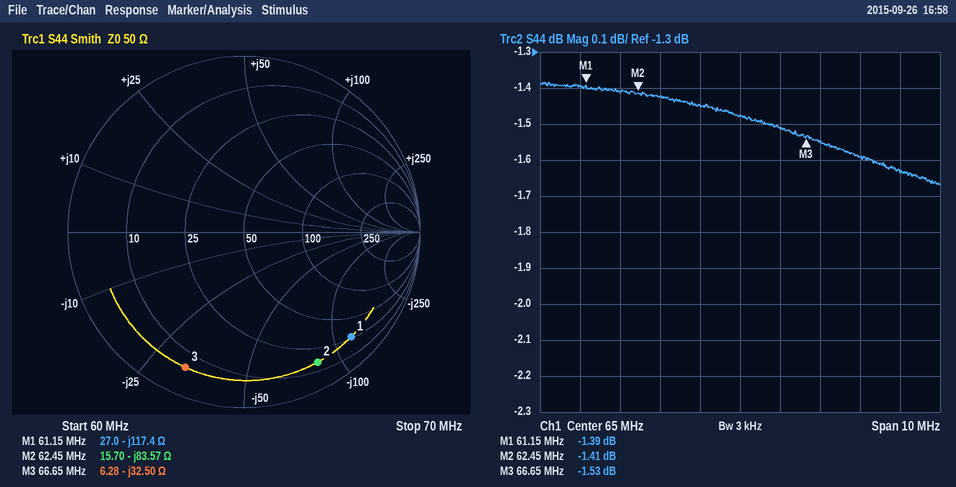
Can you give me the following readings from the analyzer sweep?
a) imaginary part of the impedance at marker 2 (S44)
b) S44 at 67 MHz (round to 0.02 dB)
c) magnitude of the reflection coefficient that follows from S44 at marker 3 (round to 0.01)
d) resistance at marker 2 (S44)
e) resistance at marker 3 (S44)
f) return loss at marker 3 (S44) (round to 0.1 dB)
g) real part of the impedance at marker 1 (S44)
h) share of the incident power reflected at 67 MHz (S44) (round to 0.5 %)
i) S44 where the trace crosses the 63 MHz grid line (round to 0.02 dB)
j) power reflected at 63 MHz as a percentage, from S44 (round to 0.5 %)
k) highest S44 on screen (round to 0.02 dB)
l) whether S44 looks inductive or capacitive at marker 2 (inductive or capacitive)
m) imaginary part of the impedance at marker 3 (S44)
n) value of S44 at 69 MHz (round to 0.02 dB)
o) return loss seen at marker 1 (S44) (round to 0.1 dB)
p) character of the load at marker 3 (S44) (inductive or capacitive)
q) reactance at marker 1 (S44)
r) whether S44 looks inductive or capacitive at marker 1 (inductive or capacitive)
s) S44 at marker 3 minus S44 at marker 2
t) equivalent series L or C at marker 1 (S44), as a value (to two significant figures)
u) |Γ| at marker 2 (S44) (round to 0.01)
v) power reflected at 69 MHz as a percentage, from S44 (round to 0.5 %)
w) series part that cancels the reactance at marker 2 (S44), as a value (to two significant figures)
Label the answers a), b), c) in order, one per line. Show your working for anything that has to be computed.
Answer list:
a) -83.57 Ω
b) -1.54 dB
c) 10^(-1.53/20) ≈ 0.84
d) 15.70 Ω
e) 6.28 Ω
f) 1.5 dB
g) 27.0 Ω
h) 10^(-1.54/10) ≈ 70.1 %, so 70.0 % to the nearest 0.5 %
i) -1.42 dB
j) 10^(-1.42/10) ≈ 72.1 %, so 72.0 % to the nearest 0.5 %
k) -1.38 dB
l) capacitive
m) -32.50 Ω
n) -1.64 dB
o) 1.4 dB
p) capacitive
q) -117.4 Ω
r) capacitive
s) -1.53 − (-1.41) = -0.12 dB
t) C = 1/(2π × 61.15 MHz × 117.4 Ω) ≈ 22 pF
u) 0.85
v) 10^(-1.64/10) ≈ 68.5 %
w) L = 83.57 Ω/(2π × 62.45 MHz) ≈ 213 nH, so 210 nH to two significant figures
